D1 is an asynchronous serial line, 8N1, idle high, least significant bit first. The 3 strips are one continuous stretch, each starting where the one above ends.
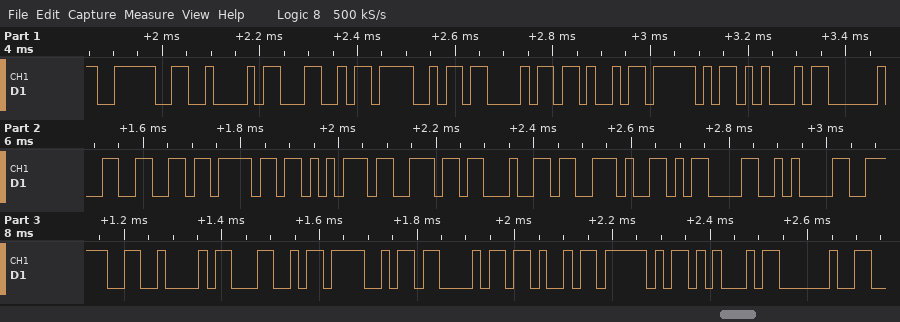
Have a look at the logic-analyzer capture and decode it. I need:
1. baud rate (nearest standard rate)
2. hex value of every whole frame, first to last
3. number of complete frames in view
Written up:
57600 baud
0x3E 0x42 0x4C 0x4F 0x43 0x4B 0x5F 0x45 0x20 0x66 0x6F 0x75 0x6E 0x64 0x2E 0x0D 0x0A 0x3E 0x42 0x4C 0x4F 0x43 0x4B 0x5F 0x45 0x20
26
